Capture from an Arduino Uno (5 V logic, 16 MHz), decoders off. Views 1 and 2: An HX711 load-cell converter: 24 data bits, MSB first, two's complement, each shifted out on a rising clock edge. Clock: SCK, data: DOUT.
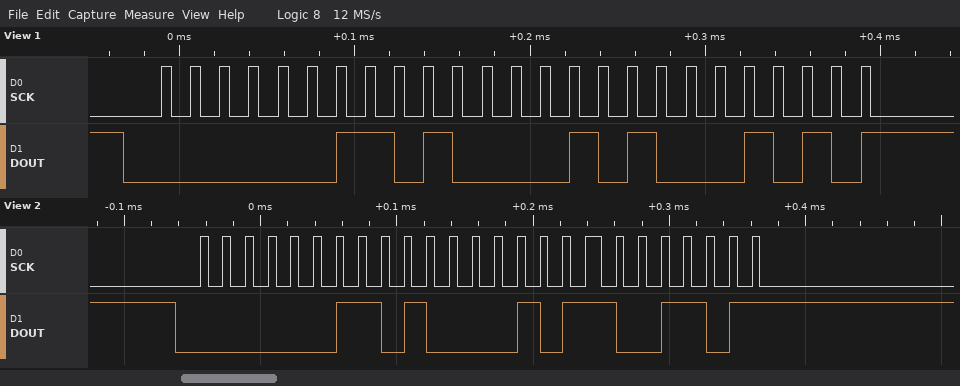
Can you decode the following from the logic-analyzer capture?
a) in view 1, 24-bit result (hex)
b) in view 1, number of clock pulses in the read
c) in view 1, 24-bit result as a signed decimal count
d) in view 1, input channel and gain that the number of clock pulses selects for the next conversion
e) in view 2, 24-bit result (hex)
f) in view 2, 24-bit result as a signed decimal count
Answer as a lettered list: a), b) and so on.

a) 0x03428A
b) 25
c) 213642
d) channel A, gain 128
e) 0x0342CD
f) 213709
